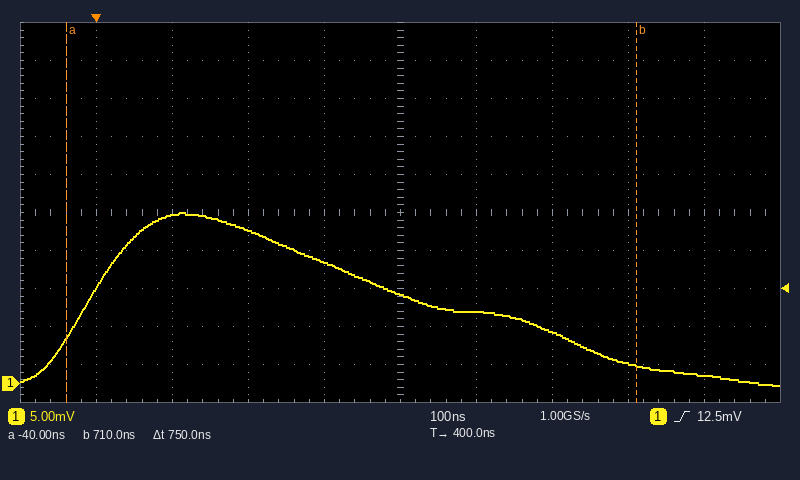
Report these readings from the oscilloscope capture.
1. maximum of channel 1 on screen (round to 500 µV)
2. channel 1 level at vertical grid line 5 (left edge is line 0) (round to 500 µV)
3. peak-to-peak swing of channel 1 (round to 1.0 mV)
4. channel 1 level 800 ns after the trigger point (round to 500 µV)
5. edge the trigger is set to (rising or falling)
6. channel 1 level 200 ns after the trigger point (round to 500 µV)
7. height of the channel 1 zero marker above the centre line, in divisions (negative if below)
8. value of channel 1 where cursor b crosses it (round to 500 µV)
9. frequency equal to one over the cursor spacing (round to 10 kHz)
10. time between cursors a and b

22.5 mV
11.5 mV
23.0 mV
1.0 mV
rising
20.0 mV
-4.5 div
2.5 mV
1.33 MHz
750 ns
